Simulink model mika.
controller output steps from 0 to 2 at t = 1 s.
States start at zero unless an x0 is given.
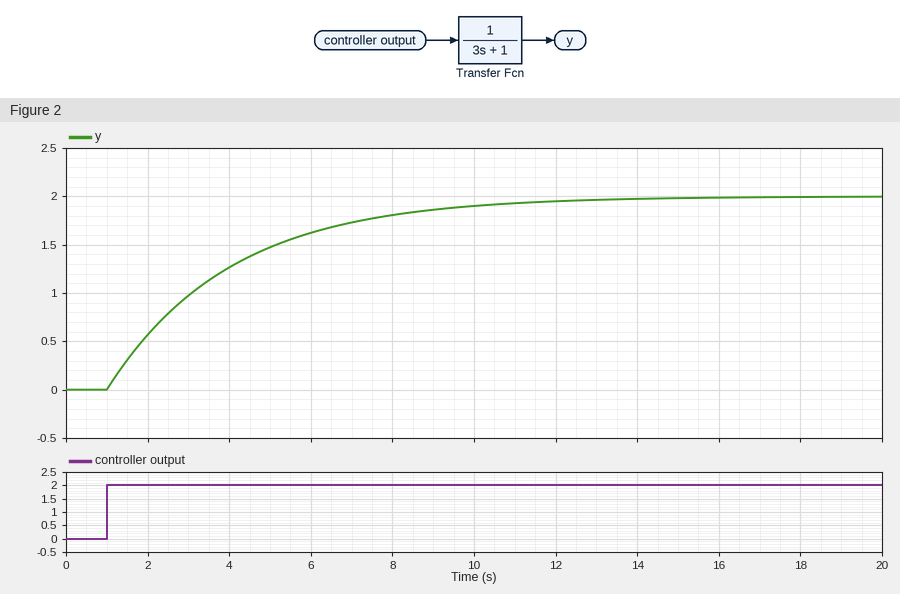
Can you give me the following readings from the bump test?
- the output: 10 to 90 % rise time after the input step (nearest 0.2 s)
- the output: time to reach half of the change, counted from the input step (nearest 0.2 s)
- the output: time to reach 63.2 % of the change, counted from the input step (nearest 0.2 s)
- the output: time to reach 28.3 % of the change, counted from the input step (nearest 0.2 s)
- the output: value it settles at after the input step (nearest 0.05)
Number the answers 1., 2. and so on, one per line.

1. 6.6 s
2. 2.0 s
3. 3.0 s
4. 1.0 s
5. 2.00
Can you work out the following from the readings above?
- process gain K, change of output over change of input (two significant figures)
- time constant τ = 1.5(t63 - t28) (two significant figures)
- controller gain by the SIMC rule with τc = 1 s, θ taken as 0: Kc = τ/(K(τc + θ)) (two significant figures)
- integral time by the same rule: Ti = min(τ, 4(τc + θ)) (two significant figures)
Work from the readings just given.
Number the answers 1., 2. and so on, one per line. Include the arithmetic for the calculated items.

1. (2 - 0) / 2 = 1.0
2. 1.5 × (3 - 1) = 3.0 s
3. 3 / (1 × (1 + 0)) = 3.0
4. min(3, 4 × (1 + 0)) = 3.0 s
